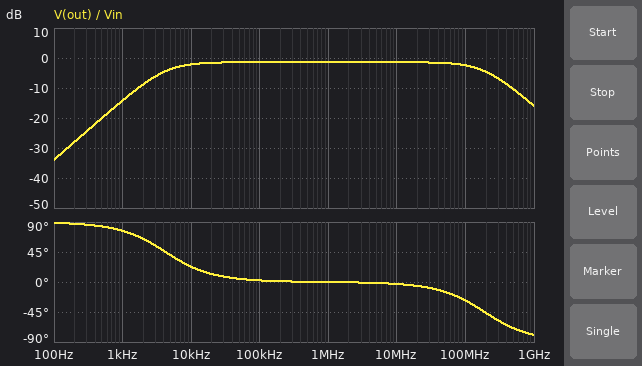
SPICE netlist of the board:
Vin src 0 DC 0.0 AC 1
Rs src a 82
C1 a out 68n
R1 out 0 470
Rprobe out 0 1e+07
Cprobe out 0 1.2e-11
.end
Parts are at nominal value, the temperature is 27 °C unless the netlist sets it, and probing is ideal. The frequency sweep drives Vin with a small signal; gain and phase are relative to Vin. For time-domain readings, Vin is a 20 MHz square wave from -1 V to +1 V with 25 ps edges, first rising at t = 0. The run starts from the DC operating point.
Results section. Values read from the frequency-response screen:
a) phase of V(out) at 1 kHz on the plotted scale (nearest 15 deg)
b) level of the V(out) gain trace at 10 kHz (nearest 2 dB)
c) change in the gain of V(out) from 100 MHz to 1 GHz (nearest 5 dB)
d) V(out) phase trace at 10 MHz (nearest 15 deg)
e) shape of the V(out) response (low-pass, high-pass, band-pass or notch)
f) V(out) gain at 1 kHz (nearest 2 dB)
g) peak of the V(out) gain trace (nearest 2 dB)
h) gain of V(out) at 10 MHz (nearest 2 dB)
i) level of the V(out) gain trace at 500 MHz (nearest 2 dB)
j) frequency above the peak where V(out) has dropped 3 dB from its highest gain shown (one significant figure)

75 deg
-2 dB
-15 dB
0 deg
band-pass
-14 dB
-2 dB
-2 dB
-10 dB
200 MHz
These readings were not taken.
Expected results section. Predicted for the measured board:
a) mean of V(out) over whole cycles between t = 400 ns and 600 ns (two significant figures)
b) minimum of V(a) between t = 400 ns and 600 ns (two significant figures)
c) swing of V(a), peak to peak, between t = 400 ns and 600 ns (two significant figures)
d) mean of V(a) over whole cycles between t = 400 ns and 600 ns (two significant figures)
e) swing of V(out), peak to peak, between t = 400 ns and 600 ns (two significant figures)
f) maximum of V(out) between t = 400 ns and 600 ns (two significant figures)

840 mV
-1.0 V
1.7 V
-150 mV
1.7 V
1.7 V
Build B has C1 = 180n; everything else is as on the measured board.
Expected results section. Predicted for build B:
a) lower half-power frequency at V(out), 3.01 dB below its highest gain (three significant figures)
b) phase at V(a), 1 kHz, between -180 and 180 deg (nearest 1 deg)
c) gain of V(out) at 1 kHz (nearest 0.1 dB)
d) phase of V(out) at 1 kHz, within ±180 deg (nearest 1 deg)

1.60 kHz
-4 deg
-6.9 dB
58 deg
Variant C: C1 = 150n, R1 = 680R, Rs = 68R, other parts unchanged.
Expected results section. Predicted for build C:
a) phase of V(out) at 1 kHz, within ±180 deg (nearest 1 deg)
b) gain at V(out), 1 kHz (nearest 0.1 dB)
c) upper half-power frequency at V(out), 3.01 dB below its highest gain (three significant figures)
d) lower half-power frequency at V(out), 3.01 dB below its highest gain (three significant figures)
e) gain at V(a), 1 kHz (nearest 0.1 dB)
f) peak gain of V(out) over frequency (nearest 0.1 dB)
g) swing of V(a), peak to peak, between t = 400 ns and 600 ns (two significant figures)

55 deg
-5.6 dB
215 MHz
1.42 kHz
-0.3 dB
-0.8 dB
1.8 V
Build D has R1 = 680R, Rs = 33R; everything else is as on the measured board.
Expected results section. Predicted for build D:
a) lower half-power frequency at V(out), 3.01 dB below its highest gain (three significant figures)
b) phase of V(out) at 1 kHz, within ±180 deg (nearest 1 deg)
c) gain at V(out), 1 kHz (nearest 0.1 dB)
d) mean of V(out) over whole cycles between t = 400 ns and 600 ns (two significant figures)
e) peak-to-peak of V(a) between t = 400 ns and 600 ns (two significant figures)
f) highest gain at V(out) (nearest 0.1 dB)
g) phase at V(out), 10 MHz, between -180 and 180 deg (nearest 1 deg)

3.28 kHz
73 deg
-11.1 dB
940 mV
1.9 V
-0.4 dB
-1 deg
